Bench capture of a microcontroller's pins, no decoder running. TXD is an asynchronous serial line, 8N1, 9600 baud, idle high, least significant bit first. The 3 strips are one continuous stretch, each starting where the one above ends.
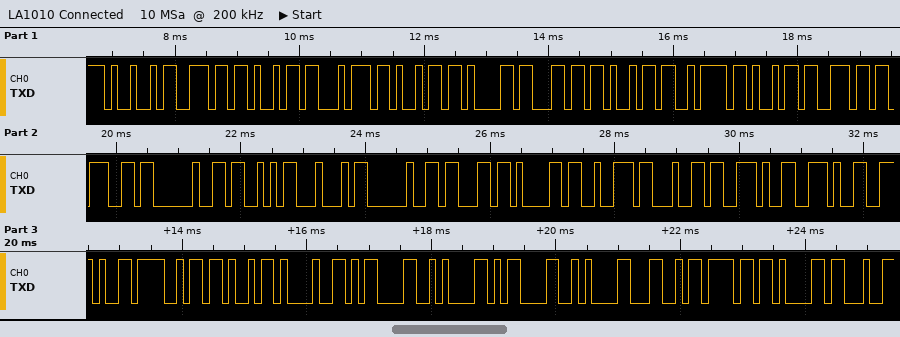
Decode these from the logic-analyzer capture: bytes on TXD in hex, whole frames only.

0x49 0x6E 0x69 0x74 0x69 0x61 0x6C 0x69 0x7A 0x69 0x6E 0x67 0x20 0x53 0x44 0x20 0x63 0x61 0x72 0x64 0x2E 0x2E 0x2E 0x4F 0x4B 0x21 0x0D 0x0A 0x0D 0x0A 0x4C 0x6F 0x61
